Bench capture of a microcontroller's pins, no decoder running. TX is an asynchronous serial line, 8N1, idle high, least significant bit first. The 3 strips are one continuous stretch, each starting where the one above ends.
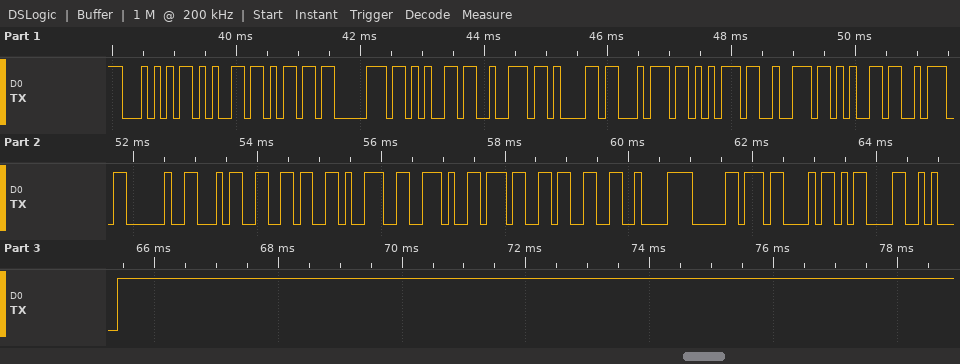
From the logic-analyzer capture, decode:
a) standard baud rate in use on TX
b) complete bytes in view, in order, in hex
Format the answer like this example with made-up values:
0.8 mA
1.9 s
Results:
9600 baud
54 65 6D 70 65 72 61 74 75 72 65 3A 20 34 36 39 2E 37 33 C2 B0 43 0D 0A
